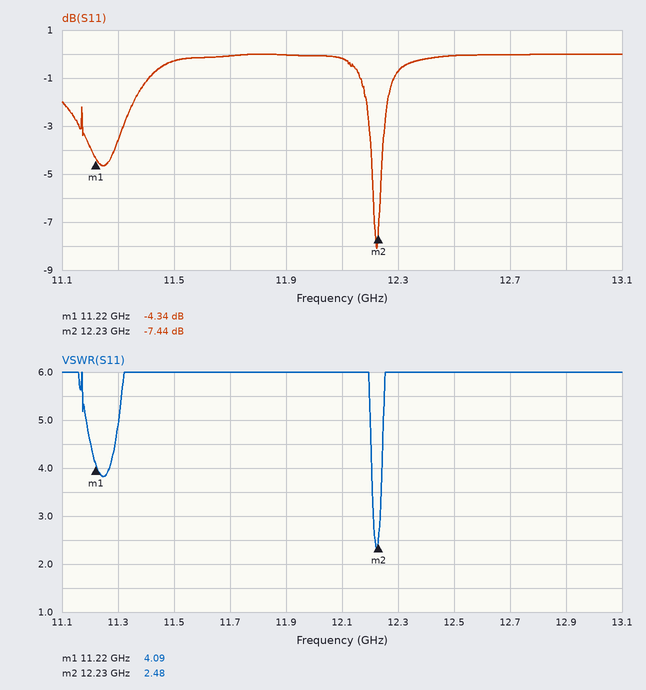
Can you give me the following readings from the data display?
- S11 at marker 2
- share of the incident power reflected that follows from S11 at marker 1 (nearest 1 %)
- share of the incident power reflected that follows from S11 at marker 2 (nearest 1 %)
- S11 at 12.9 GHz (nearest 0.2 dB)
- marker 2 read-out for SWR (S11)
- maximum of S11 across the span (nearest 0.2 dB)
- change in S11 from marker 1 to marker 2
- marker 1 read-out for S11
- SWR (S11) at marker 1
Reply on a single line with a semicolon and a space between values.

-7.44 dB; 37 %; 18 %; 0.0 dB; 2.48; 0.0 dB; -3.10 dB; -4.34 dB; 4.09
